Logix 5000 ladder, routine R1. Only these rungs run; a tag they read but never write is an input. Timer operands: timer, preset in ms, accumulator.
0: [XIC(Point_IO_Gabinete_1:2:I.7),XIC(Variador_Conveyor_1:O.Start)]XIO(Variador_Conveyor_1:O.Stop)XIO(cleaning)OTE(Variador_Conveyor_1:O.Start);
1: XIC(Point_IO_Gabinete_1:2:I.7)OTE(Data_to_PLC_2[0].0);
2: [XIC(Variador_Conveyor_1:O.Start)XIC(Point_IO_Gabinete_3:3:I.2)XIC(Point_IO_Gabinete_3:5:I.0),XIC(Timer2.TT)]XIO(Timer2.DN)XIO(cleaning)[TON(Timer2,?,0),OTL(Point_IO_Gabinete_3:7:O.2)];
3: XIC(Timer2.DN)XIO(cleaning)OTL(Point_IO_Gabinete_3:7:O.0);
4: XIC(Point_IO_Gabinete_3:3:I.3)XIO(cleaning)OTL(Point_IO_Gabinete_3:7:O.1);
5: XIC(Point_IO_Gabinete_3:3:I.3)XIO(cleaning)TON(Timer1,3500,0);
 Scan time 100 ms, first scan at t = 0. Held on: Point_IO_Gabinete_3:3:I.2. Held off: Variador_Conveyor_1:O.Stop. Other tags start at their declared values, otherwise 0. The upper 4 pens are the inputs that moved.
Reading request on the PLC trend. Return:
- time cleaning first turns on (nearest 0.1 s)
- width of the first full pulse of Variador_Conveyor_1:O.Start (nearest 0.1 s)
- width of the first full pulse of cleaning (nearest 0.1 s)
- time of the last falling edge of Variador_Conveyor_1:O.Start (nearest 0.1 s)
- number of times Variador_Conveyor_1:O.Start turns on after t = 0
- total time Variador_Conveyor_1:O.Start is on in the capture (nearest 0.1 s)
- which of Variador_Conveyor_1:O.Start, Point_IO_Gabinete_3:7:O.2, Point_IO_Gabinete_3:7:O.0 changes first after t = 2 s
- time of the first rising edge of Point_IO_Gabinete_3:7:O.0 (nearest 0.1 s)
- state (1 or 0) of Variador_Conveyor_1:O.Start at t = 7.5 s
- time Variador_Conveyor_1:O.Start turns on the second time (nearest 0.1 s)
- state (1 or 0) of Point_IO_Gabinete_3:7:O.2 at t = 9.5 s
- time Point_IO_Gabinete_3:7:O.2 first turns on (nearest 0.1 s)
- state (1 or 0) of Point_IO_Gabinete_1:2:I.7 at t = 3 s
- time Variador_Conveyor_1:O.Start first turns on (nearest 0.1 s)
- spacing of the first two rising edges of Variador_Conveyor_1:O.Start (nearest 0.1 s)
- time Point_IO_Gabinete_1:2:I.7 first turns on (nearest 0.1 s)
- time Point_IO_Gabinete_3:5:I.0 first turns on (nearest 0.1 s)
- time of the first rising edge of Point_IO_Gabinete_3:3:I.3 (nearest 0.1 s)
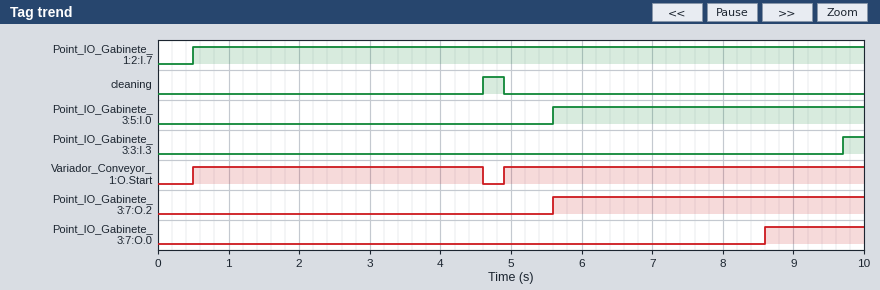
4.6 s
4.1 s
0.3 s
4.6 s
2
9.2 s
Variador_Conveyor_1:O.Start
8.6 s
1
4.9 s
1
5.6 s
1
0.5 s
4.4 s
0.5 s
5.6 s
9.7 s
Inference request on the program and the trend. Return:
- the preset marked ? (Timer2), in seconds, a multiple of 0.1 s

3.0 s
